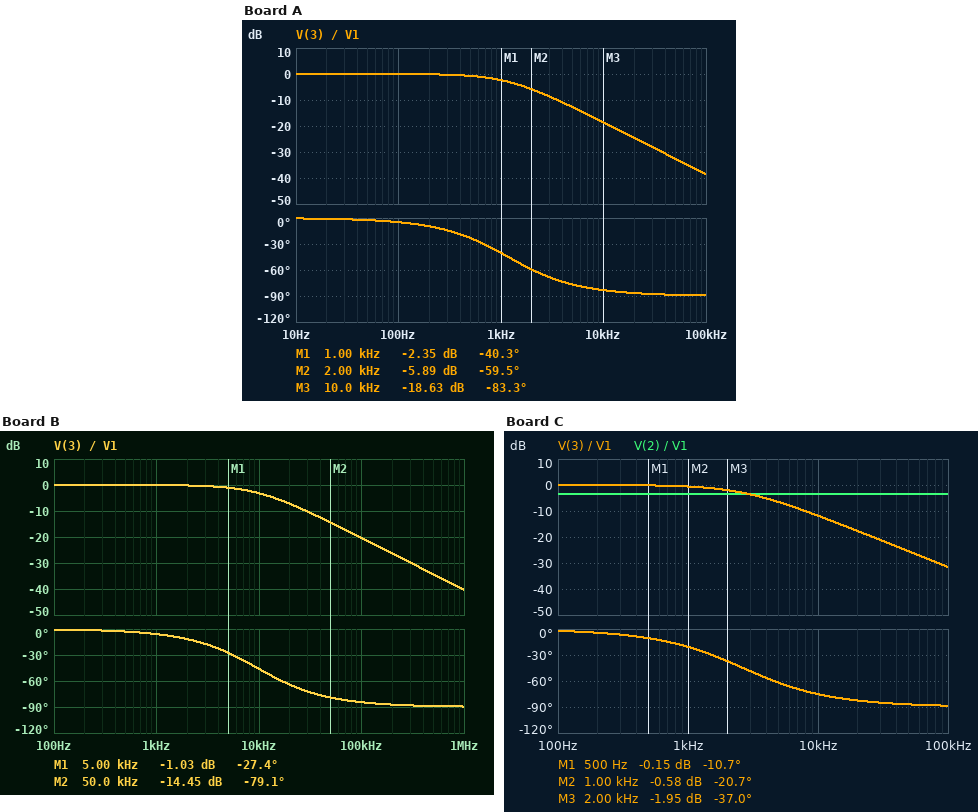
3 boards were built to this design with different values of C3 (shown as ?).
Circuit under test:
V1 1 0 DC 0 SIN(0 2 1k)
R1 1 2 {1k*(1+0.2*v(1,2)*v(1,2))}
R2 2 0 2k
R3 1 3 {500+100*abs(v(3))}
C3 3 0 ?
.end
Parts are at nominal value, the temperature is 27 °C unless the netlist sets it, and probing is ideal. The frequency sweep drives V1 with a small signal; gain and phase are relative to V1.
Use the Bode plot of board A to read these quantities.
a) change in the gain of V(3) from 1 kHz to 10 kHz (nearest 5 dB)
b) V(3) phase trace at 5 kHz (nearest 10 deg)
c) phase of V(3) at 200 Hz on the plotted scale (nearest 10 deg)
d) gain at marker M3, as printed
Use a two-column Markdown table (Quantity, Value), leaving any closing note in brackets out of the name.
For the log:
| Quantity | Value |
|---|---|
| change in the gain of V(3) from 1 kHz to 10 kHz | -15 dB |
| V(3) phase trace at 5 kHz | -80 deg |
| phase of V(3) at 200 Hz on the plotted scale | -10 deg |
| gain at marker M3, as printed | -18.63 dB |
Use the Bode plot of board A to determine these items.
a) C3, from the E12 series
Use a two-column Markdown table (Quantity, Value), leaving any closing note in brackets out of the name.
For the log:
| Quantity | Value |
|---|---|
| C3, from the E12 series | 270 nF |
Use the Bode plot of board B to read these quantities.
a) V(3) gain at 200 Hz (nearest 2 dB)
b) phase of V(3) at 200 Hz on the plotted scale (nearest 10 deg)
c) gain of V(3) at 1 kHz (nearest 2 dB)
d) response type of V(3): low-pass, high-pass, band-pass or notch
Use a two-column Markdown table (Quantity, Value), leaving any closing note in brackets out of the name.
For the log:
| Quantity | Value |
|---|---|
| V(3) gain at 200 Hz | 0 dB |
| phase of V(3) at 200 Hz on the plotted scale | 0 deg |
| gain of V(3) at 1 kHz | 0 dB |
| response type of V(3): low-pass, high-pass, band-pass or notch | low-pass |
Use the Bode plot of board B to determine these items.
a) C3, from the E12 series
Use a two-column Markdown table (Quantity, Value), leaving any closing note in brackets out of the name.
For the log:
| Quantity | Value |
|---|---|
| C3, from the E12 series | 33 nF |
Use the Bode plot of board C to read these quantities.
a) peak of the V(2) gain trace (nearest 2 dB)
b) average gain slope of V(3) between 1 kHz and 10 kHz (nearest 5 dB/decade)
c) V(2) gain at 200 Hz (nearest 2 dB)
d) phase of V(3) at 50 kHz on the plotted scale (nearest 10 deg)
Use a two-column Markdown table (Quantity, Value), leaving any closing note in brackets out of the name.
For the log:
| Quantity | Value |
|---|---|
| peak of the V(2) gain trace | -4 dB |
| average gain slope of V(3) between 1 kHz and 10 kHz | -10 dB/decade |
| V(2) gain at 200 Hz | -4 dB |
| phase of V(3) at 50 kHz on the plotted scale | -90 deg |
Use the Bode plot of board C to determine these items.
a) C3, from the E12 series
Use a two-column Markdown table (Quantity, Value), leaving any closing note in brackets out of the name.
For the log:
| Quantity | Value |
|---|---|
| C3, from the E12 series | 120 nF |
